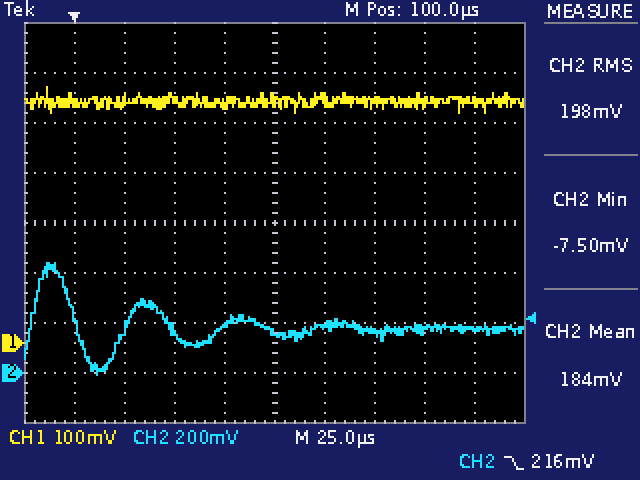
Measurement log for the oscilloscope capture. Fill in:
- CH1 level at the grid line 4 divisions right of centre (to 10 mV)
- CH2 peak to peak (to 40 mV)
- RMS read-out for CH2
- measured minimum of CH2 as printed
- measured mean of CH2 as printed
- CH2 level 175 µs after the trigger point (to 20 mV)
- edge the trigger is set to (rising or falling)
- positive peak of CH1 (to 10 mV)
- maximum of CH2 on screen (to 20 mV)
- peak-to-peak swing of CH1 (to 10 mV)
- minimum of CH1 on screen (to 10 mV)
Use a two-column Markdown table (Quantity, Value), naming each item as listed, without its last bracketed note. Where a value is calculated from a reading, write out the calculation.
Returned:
| Quantity | Value |
|---|---|
| CH1 level at the grid line 4 divisions right of centre | 480 mV |
| CH2 peak to peak | 440 mV |
| RMS read-out for CH2 | 198 mV |
| measured minimum of CH2 as printed | -7.50 mV |
| measured mean of CH2 as printed | 184 mV |
| CH2 level 175 µs after the trigger point | 180 mV |
| edge the trigger is set to | falling |
| positive peak of CH1 | 510 mV |
| maximum of CH2 on screen | 440 mV |
| peak-to-peak swing of CH1 | 510 mV − (460 mV) = 50 mV |
| minimum of CH1 on screen | 460 mV |
